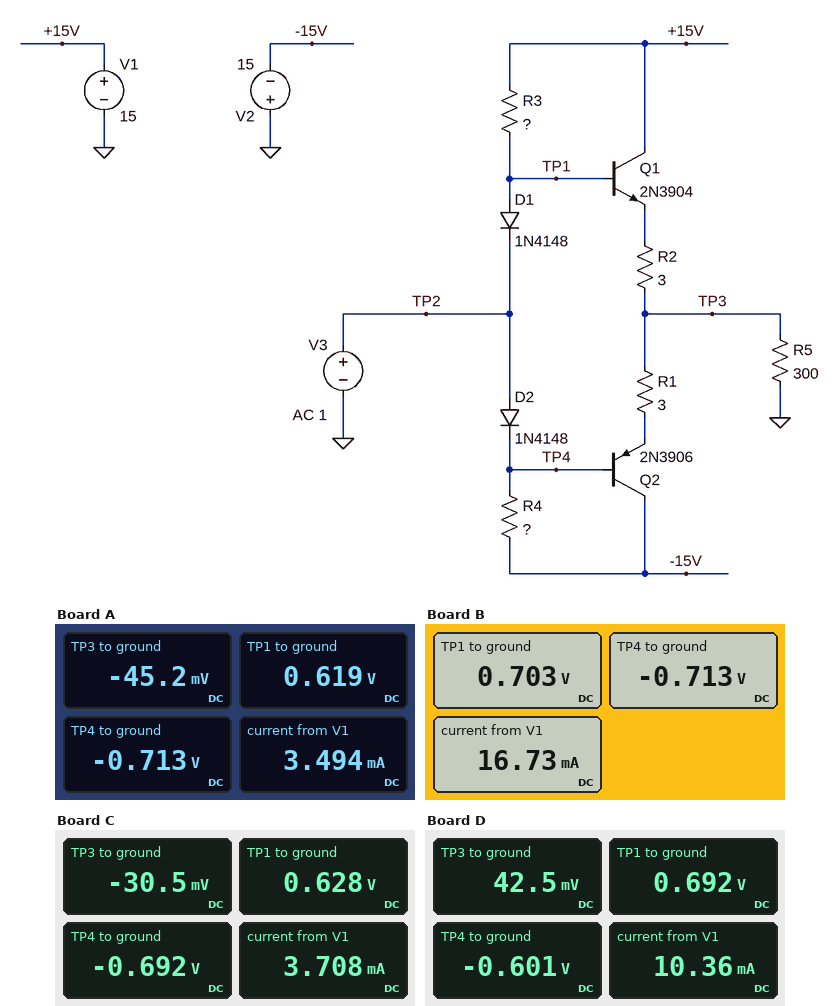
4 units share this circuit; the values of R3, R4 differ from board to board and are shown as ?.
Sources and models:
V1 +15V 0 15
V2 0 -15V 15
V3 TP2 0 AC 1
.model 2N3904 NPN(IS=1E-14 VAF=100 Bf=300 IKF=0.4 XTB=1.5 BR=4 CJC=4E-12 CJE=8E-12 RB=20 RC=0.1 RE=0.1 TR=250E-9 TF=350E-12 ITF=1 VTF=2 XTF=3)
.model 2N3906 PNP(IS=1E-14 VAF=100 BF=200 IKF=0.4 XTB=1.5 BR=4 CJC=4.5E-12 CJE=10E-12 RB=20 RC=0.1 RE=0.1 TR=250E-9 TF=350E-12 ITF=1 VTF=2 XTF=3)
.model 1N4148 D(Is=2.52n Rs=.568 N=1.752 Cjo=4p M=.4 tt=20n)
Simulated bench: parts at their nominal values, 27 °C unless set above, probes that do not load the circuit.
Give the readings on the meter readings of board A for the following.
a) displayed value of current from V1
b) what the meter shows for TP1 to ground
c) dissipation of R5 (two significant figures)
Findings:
3.494 mA
0.619 V
6.8 µW
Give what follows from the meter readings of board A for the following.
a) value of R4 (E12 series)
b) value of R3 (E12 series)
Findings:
1 kΩ
6.8 kΩ
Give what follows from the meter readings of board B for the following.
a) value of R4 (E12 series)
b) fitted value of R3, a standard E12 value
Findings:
1 kΩ
1.2 kΩ
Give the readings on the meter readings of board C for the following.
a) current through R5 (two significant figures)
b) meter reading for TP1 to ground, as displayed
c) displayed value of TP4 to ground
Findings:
100 µA
0.628 V
-0.692 V
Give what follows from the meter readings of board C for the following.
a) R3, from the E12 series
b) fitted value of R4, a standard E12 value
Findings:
5.6 kΩ
1.5 kΩ
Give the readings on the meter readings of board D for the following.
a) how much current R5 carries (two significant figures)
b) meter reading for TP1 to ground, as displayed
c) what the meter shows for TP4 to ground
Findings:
140 µA
0.692 V
-0.601 V
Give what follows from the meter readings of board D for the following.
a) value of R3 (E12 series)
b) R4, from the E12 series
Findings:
1.5 kΩ
10 kΩ
